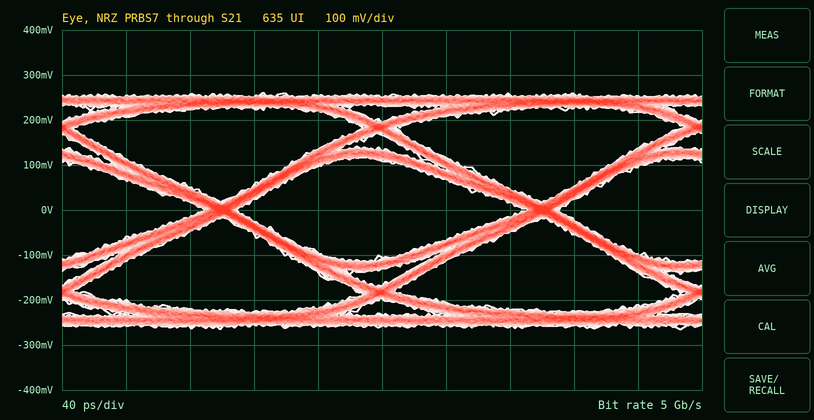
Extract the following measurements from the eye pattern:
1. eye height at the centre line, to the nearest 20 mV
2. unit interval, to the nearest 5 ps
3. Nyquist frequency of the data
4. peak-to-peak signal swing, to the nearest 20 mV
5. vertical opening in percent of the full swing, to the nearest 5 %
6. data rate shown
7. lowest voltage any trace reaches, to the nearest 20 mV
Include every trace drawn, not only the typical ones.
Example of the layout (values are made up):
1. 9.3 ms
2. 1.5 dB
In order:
1. 220 mV
2. 200 ps
3. 2.5 GHz
4. 520 mV
5. 40 %
6. 5 Gb/s
7. -260 mV
